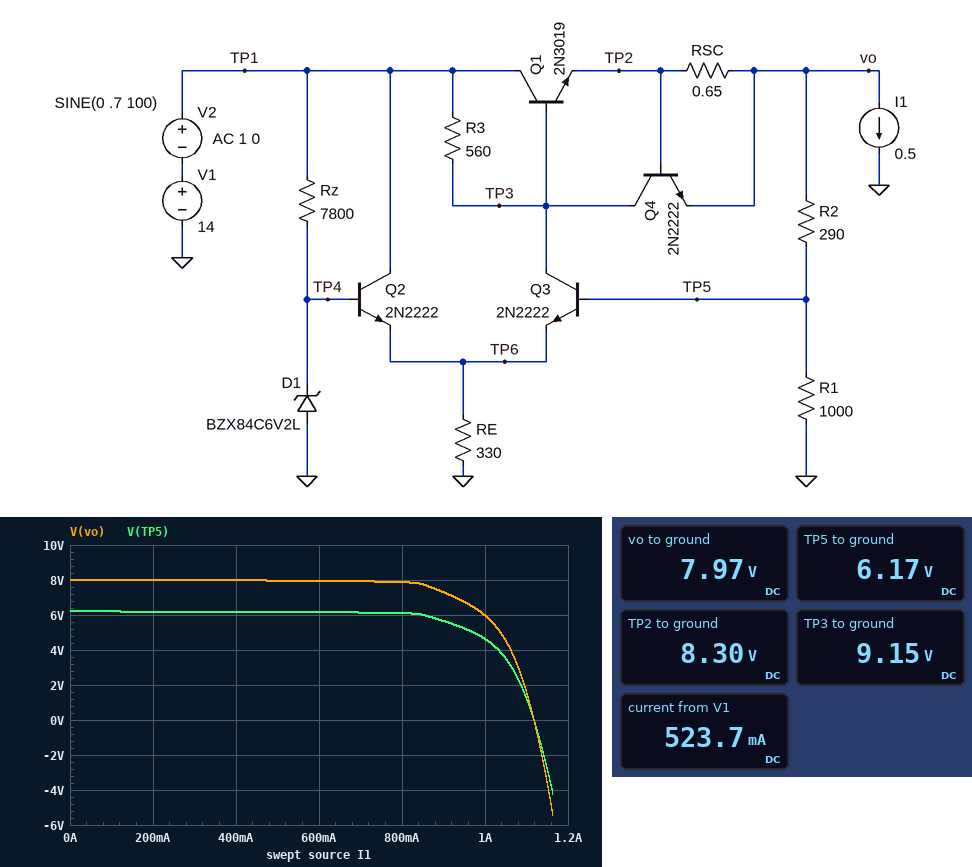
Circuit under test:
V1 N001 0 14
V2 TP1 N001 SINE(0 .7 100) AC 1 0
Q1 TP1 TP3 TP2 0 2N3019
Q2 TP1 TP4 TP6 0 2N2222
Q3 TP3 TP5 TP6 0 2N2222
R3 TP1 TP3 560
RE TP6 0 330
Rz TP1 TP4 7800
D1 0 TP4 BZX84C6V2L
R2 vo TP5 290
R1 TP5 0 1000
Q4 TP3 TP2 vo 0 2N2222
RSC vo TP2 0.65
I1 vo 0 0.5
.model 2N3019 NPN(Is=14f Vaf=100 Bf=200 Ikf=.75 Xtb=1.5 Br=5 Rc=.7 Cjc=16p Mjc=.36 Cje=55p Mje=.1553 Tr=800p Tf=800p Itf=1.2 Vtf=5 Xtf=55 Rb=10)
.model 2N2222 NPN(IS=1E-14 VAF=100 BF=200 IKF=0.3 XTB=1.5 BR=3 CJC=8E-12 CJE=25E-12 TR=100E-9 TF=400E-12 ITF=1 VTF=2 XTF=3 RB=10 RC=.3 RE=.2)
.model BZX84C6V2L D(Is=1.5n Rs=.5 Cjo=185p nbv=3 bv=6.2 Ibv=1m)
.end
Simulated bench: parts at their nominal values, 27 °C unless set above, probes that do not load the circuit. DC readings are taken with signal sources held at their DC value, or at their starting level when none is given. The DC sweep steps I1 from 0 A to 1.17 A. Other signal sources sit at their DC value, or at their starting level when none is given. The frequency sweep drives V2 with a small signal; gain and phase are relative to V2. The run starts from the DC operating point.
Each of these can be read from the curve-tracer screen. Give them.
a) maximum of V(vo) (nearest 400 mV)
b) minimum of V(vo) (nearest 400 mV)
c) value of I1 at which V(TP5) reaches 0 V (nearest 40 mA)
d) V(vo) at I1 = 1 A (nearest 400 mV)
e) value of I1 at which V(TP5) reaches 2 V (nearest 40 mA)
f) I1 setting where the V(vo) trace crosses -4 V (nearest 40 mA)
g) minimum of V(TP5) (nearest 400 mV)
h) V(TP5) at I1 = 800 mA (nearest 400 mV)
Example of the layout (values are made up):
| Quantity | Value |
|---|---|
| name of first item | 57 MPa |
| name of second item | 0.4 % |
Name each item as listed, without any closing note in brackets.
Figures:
| Quantity | Value |
|---|---|
| maximum of V(vo) | 8.0 V |
| minimum of V(vo) | -5.6 V |
| value of I1 at which V(TP5) reaches 0 V | 1.12 A |
| V(vo) at I1 = 1 A | 6.0 V |
| value of I1 at which V(TP5) reaches 2 V | 1.08 A |
| I1 setting where the V(vo) trace crosses -4 V | 1.16 A |
| minimum of V(TP5) | -4.4 V |
| V(TP5) at I1 = 800 mA | 6.0 V |
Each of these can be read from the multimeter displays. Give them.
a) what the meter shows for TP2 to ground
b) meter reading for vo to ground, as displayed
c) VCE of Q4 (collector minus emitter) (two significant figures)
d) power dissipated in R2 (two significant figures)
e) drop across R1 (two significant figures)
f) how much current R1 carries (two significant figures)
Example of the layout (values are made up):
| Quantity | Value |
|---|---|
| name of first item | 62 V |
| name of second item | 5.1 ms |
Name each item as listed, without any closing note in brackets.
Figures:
| Quantity | Value |
|---|---|
| what the meter shows for TP2 to ground | 8.30 V |
| meter reading for vo to ground, as displayed | 7.97 V |
| VCE of Q4 (collector minus emitter) | 1.2 V |
| power dissipated in R2 | 11 mW |
| drop across R1 | 6.2 V |
| how much current R1 carries | 6.2 mA |
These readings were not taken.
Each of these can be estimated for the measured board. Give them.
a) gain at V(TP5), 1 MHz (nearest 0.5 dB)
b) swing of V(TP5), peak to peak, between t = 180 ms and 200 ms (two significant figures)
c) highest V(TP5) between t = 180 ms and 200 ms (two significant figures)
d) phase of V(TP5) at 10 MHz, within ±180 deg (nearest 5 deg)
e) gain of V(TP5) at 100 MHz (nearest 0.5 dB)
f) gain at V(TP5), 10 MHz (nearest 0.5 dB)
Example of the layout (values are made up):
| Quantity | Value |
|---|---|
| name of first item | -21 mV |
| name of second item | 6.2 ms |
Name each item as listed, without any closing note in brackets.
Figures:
| Quantity | Value |
|---|---|
| gain at V(TP5), 1 MHz | -30.0 dB |
| swing of V(TP5), peak to peak, between t = 180 ms and 200 ms | 37 mV |
| highest V(TP5) between t = 180 ms and 200 ms | 6.2 V |
| phase of V(TP5) at 10 MHz, within ±180 deg | 45 deg |
| gain of V(TP5) at 100 MHz | -15.5 dB |
| gain at V(TP5), 10 MHz | -15.0 dB |
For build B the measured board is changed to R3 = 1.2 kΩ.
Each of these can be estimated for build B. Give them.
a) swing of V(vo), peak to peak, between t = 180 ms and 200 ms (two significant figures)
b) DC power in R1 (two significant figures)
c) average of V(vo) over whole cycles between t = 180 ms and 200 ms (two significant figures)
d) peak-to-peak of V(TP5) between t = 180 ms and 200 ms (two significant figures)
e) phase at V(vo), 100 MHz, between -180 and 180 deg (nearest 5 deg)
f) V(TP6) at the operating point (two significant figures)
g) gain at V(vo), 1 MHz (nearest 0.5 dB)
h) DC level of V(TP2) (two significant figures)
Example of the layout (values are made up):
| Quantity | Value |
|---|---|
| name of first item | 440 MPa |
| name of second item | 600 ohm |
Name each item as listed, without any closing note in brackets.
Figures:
| Quantity | Value |
|---|---|
| swing of V(vo), peak to peak, between t = 180 ms and 200 ms | 510 mV |
| DC power in R1 | 37 mW |
| average of V(vo) over whole cycles between t = 180 ms and 200 ms | 7.7 V |
| peak-to-peak of V(TP5) between t = 180 ms and 200 ms | 400 mV |
| phase at V(vo), 100 MHz, between -180 and 180 deg | 0 deg |
| V(TP6) at the operating point | 5.5 V |
| gain at V(vo), 1 MHz | -10.5 dB |
| DC level of V(TP2) | 8.2 V |
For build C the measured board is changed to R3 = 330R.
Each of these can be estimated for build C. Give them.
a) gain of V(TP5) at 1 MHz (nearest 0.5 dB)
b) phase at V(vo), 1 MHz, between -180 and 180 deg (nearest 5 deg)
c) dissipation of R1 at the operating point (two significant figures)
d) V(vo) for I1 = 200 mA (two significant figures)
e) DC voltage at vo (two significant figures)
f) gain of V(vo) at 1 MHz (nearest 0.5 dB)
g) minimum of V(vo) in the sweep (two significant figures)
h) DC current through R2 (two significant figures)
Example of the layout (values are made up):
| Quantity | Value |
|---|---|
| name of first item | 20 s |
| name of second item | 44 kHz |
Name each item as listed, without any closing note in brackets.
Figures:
| Quantity | Value |
|---|---|
| gain of V(TP5) at 1 MHz | -28.5 dB |
| phase at V(vo), 1 MHz, between -180 and 180 deg | 30 deg |
| dissipation of R1 at the operating point | 39 mW |
| V(vo) for I1 = 200 mA | 8.1 V |
| DC voltage at vo | 8.0 V |
| gain of V(vo) at 1 MHz | -25.5 dB |
| minimum of V(vo) in the sweep | 880 mV |
| DC current through R2 | 6.3 mA |
